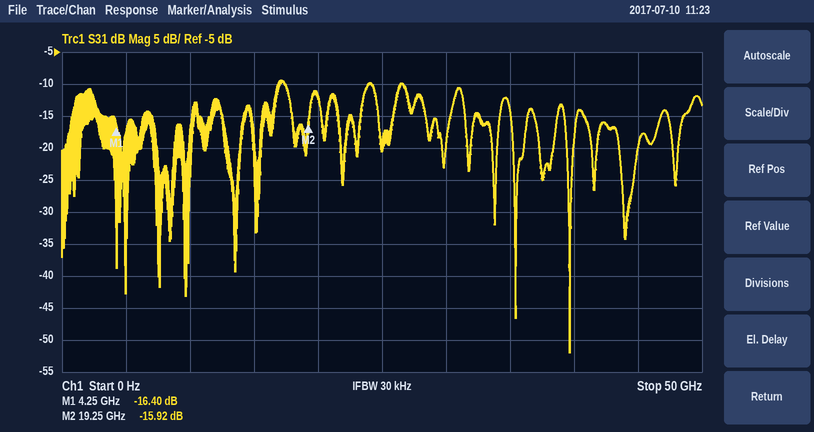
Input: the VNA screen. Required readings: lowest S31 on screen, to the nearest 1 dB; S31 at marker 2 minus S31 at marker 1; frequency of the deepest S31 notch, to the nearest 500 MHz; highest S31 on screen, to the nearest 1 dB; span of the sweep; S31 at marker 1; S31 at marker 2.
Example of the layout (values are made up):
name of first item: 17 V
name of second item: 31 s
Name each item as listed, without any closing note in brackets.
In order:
lowest S31 on screen, to the nearest 1 dB: -52 dB
S31 at marker 2 minus S31 at marker 1: 0.48 dB
frequency of the deepest S31 notch, to the nearest 500 MHz: 39.5 GHz
highest S31 on screen, to the nearest 1 dB: -9 dB
span of the sweep: 50 GHz
S31 at marker 1: -16.40 dB
S31 at marker 2: -15.92 dB
